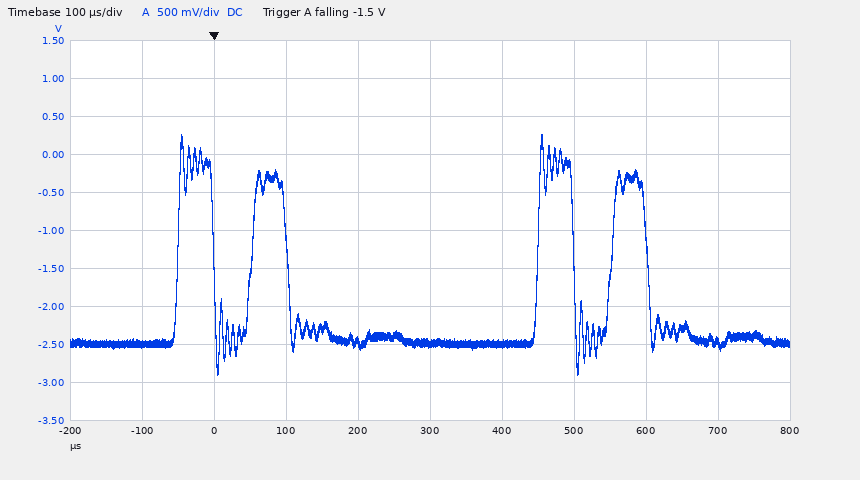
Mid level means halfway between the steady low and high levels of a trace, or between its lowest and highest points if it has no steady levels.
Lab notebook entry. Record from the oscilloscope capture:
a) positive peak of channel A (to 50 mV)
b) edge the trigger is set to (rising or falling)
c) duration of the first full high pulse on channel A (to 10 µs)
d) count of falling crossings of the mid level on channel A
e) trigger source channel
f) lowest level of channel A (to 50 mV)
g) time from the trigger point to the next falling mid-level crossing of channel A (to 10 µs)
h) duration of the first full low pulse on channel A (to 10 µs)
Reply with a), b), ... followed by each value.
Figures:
a) 250 mV
b) falling
c) 50 µs
d) 4
e) channel A
f) -2.90 V
g) 100 µs
h) 50 µs
